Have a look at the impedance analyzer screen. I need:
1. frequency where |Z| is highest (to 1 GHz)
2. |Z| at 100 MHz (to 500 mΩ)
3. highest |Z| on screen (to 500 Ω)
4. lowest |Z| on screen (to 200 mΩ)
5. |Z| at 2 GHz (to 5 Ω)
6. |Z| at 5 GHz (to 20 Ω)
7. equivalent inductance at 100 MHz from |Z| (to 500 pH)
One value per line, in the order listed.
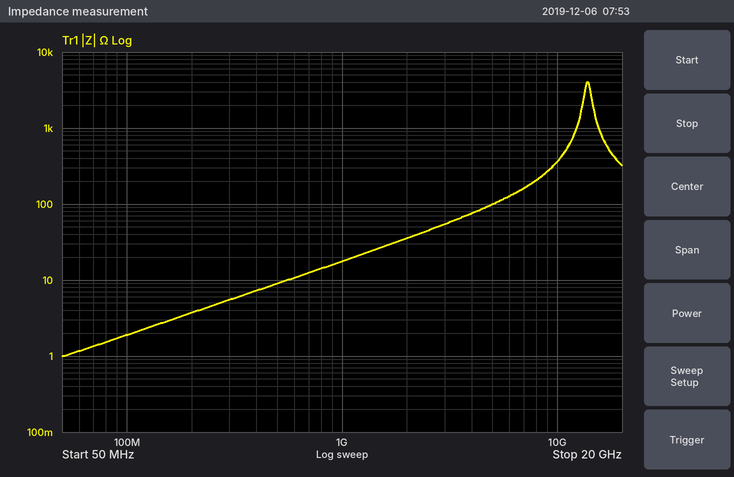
14 GHz
2.0 Ω
4.0 kΩ
1.0 Ω
35 Ω
100 Ω
3.0 nH
